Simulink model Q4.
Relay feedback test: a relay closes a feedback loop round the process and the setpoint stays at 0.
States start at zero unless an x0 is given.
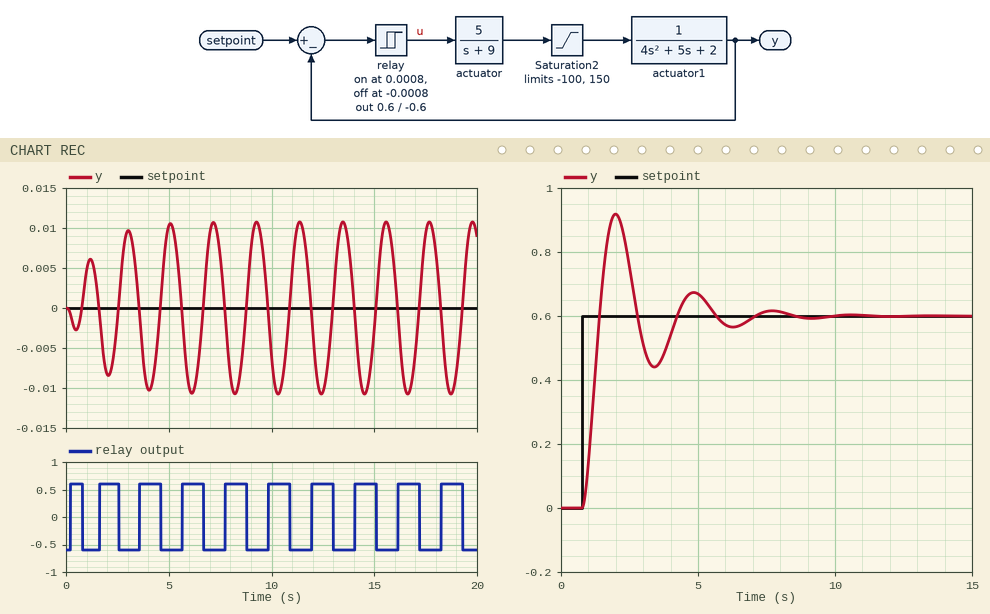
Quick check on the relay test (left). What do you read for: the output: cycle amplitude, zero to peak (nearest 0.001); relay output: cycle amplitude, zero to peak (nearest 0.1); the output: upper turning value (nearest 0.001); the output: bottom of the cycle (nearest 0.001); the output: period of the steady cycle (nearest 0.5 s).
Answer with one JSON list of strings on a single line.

["0.011", "0.6", "0.011", "-0.011", "2.0 s"]
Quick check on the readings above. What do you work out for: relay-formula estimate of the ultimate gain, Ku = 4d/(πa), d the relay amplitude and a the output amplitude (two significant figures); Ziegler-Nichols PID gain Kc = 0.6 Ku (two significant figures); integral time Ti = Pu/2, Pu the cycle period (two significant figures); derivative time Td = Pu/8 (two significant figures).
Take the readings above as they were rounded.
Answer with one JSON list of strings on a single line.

["69", "41", "1.0 s", "0.25 s"]
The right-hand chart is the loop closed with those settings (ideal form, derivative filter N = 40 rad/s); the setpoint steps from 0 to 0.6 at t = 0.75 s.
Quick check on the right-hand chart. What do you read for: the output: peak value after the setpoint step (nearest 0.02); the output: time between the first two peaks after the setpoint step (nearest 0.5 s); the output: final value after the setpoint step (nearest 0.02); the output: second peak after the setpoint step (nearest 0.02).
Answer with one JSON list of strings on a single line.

["0.92", "3.0 s", "0.60", "0.68"]
